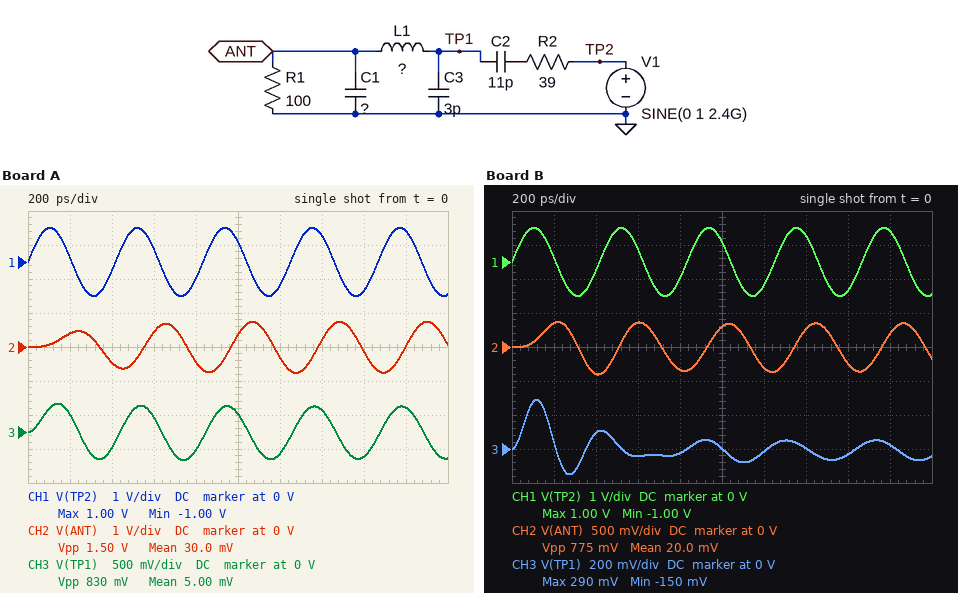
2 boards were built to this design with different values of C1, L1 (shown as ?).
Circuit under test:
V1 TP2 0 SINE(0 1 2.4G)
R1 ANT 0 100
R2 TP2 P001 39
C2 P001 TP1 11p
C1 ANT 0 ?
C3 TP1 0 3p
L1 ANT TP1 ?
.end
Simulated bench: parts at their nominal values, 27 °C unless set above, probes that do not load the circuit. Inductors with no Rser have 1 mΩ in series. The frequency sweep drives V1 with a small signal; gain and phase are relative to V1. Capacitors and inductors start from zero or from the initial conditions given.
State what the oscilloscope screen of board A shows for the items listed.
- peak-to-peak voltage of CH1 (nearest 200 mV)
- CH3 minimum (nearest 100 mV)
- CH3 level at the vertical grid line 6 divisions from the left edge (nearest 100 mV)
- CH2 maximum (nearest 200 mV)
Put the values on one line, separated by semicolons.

2.0 V; -400 mV; -300 mV; 800 mV
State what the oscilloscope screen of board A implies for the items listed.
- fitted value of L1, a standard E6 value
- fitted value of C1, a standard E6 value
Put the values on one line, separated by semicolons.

3.3 nH; 1.5 pF
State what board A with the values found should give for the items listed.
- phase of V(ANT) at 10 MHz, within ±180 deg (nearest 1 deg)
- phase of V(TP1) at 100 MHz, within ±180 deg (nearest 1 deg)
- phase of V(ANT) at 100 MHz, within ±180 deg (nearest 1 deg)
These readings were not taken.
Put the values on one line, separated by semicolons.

83 deg; 37 deg; 36 deg
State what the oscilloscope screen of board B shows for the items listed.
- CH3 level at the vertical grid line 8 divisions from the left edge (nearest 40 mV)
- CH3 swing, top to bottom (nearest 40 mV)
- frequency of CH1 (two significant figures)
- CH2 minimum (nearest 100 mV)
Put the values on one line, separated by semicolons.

-40 mV; 440 mV; 2.4 GHz; -400 mV
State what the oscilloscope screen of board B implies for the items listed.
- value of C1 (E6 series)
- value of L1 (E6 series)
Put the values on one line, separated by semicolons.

4.7 pF; 1 nH
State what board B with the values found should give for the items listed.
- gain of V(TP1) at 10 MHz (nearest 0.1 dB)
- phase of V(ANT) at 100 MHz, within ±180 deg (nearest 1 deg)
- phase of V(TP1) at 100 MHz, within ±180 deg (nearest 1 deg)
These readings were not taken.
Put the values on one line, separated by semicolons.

-23.3 dB; 31 deg; 31 deg
